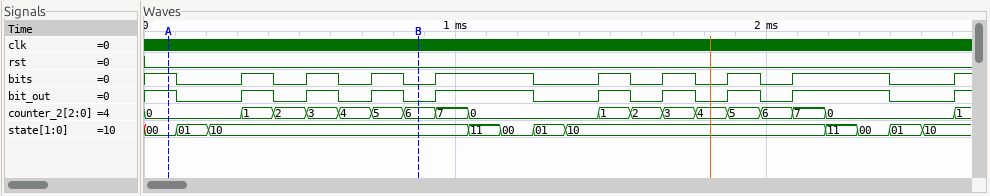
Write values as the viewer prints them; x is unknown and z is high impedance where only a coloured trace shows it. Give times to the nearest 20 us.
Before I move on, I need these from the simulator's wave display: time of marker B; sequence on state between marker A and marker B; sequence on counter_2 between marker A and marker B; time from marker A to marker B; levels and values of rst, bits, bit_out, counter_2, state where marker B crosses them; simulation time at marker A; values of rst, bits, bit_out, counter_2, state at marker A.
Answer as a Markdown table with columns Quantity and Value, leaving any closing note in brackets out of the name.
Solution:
| Quantity | Value |
|---|---|
| time of marker B | 880 us |
| sequence on state between marker A and marker B | 00, 01, 10 |
| sequence on counter_2 between marker A and marker B | 0, 1, 2, 3, 4, 5, 6 |
| time from marker A to marker B | 800 us |
| levels and values of rst, bits, bit_out, counter_2, state where marker B crosses them | rst=0, bits=0, bit_out=0, counter_2=6, state=10 |
| simulation time at marker A | 80 us |
| values of rst, bits, bit_out, counter_2, state at marker A | rst=0, bits=1, bit_out=1, counter_2=0, state=00 |
